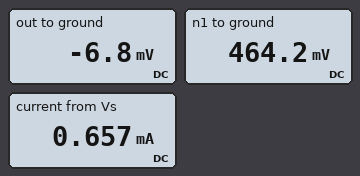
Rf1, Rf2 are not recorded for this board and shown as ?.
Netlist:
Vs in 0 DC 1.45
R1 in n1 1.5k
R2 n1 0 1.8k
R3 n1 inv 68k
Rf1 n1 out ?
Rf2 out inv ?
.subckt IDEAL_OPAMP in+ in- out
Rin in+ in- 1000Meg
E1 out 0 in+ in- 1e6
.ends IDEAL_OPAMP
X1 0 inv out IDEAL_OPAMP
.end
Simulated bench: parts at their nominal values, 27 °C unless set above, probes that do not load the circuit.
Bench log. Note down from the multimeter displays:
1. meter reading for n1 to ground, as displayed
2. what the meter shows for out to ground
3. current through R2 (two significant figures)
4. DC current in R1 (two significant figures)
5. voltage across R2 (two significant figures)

464.2 mV
-6.8 mV
260 µA
660 µA
460 mV
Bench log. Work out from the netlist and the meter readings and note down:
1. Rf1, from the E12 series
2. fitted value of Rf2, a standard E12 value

1.2 kΩ
1 kΩ
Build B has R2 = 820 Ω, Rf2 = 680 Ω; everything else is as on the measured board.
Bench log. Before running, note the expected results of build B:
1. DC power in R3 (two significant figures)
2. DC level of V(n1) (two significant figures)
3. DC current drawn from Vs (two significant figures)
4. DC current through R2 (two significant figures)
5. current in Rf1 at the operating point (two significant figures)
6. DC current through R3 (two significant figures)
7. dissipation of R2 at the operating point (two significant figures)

1.8 µW
350 mV
730 µA
430 µA
300 µA
5.2 µA
150 µW
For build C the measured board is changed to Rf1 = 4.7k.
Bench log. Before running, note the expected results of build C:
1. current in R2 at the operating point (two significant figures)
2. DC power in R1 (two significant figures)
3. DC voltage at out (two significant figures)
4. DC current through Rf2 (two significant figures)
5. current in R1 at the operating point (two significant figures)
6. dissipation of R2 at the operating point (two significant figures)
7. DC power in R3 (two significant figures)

370 µA
410 µW
-9.8 mV
9.8 µA
520 µA
250 µW
6.5 µW
